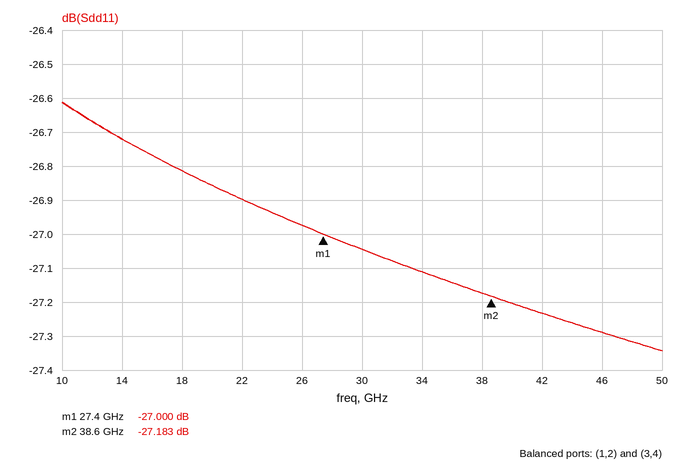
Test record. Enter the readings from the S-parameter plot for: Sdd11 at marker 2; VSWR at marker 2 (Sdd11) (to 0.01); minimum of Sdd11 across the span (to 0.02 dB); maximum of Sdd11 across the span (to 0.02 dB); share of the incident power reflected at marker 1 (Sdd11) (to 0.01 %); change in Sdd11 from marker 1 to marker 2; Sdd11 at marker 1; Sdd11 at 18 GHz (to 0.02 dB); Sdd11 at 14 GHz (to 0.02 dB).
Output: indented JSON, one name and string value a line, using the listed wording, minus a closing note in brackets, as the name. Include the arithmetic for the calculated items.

{
  "Sdd11 at marker 2": "-27.183 dB",
  "VSWR at marker 2 (Sdd11)": "(1 + 0.0437)/(1 − 0.0437) ≈ 1.09",
  "minimum of Sdd11 across the span": "-27.34 dB",
  "maximum of Sdd11 across the span": "-26.62 dB",
  "share of the incident power reflected at marker 1 (Sdd11)": "10^(-27/10) ≈ 0.20 %",
  "change in Sdd11 from marker 1 to marker 2": "-27.183 − (-27) = -0.183 dB",
  "Sdd11 at marker 1": "-27.000 dB",
  "Sdd11 at 18 GHz": "-26.82 dB",
  "Sdd11 at 14 GHz": "-26.72 dB"
}
